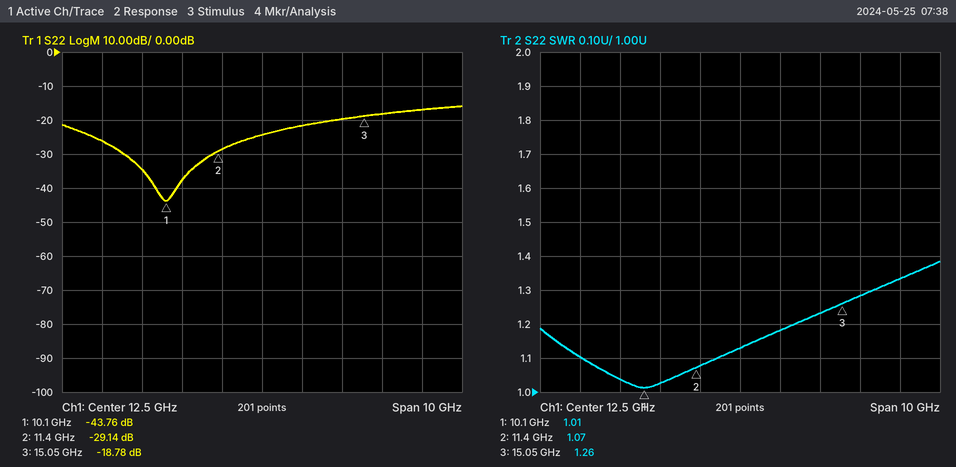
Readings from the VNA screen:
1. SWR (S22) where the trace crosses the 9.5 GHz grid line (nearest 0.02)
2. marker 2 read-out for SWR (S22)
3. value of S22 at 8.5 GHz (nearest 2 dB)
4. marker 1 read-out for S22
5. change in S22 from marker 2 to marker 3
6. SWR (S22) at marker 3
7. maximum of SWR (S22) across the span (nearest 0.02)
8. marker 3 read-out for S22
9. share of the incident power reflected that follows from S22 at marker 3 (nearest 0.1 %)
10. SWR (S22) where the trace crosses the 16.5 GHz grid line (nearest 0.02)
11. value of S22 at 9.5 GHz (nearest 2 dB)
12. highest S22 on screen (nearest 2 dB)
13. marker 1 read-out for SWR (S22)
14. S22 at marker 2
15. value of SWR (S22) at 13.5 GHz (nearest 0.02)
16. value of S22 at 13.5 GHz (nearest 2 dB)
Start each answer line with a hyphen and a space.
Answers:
- 1.04
- 1.07
- -26 dB
- -43.76 dB
- 10.36 dB
- 1.26
- 1.38
- -18.78 dB
- 1.3 %
- 1.34
- -34 dB
- -16 dB
- 1.01
- -29.14 dB
- 1.18
- -22 dB
